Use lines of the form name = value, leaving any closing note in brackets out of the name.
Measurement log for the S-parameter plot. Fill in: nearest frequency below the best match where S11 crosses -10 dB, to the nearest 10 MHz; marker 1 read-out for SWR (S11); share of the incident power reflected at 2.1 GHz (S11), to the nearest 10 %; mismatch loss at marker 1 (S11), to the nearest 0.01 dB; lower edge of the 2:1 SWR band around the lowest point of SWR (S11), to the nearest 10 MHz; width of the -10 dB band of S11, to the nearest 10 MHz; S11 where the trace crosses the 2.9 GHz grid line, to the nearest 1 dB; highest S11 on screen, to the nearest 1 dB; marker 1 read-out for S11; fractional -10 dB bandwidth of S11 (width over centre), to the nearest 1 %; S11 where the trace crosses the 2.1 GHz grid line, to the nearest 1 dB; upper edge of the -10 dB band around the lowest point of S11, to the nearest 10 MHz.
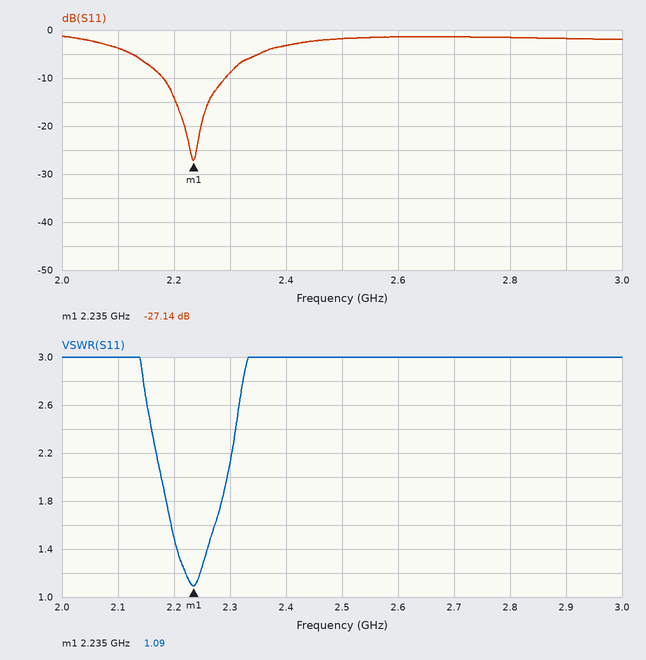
nearest frequency below the best match where S11 crosses -10 dB, to the nearest 10 MHz = 2.18 GHz
marker 1 read-out for SWR = 1.09
share of the incident power reflected at 2.1 GHz (S11), to the nearest 10 % = 40 %
mismatch loss at marker 1 (S11), to the nearest 0.01 dB = 0.01 dB
lower edge of the 2:1 SWR band around the lowest point of SWR (S11), to the nearest 10 MHz = 2.18 GHz
width of the -10 dB band of S11, to the nearest 10 MHz = 110 MHz
S11 where the trace crosses the 2.9 GHz grid line, to the nearest 1 dB = -2 dB
highest S11 on screen, to the nearest 1 dB = -1 dB
marker 1 read-out for S11 = -27.14 dB
fractional -10 dB bandwidth of S11 (width over centre), to the nearest 1 % = 5 %
S11 where the trace crosses the 2.1 GHz grid line, to the nearest 1 dB = -4 dB
upper edge of the -10 dB band around the lowest point of S11, to the nearest 10 MHz = 2.29 GHz
